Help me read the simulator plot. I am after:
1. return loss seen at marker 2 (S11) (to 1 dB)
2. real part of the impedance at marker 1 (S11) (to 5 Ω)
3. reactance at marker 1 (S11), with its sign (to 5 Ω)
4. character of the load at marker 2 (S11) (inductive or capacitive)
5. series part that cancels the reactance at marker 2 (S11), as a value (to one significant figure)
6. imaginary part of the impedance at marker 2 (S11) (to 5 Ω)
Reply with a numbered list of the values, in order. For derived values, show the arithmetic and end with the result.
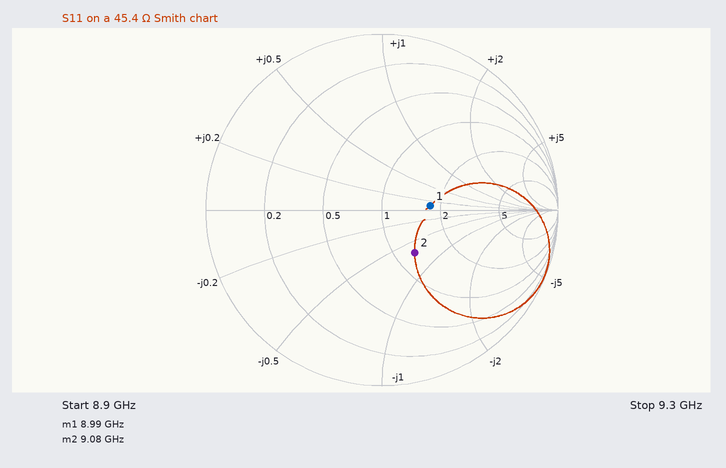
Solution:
1. 10 dB
2. 80 Ω
3. +5 Ω
4. capacitive
5. L = 30 Ω/(2π × 9.08 GHz) ≈ 526 pH, so 500 pH to one significant figure
6. -30 Ω
